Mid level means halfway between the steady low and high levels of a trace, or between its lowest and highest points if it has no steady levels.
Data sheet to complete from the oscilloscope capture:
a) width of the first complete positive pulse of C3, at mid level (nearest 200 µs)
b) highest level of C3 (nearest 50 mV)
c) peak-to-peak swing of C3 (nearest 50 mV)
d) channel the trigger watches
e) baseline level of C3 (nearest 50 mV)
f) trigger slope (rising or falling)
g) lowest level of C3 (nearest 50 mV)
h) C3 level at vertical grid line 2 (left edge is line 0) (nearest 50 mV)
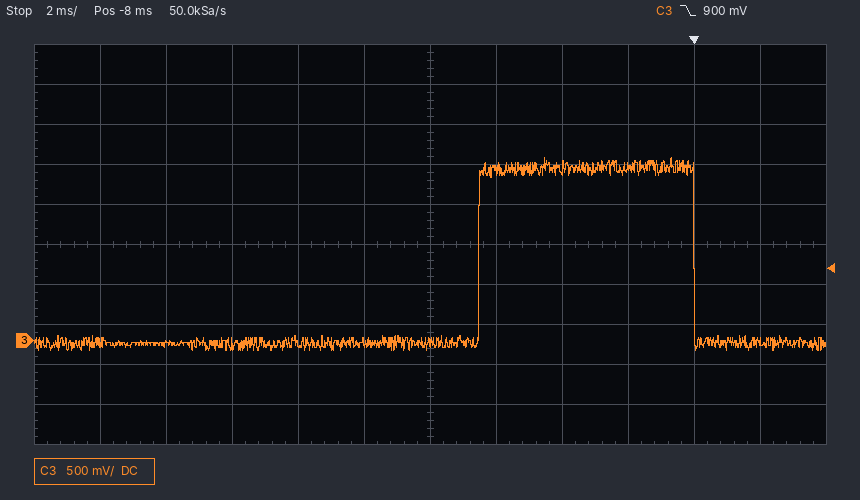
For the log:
6.6 ms
2.30 V
2.40 V
C3
-50 mV
falling
-100 mV
-50 mV
